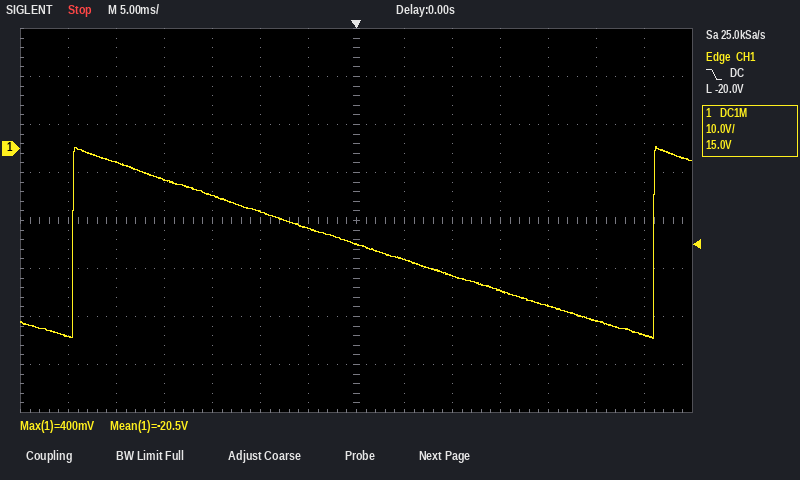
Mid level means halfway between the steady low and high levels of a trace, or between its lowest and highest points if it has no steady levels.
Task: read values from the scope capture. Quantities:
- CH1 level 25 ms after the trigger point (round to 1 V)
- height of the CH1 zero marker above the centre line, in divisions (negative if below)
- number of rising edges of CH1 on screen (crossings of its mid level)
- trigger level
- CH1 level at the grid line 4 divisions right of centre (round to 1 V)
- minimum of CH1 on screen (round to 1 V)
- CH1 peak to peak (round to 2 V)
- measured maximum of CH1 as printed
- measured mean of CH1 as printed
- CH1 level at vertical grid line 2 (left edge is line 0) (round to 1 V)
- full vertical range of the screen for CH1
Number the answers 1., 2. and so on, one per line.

1. -36 V
2. +1.5 div
3. 2
4. -20.0 V
5. -33 V
6. -40 V
7. 40 V
8. 400 mV
9. -20.5 V
10. -3 V
11. 80 V
